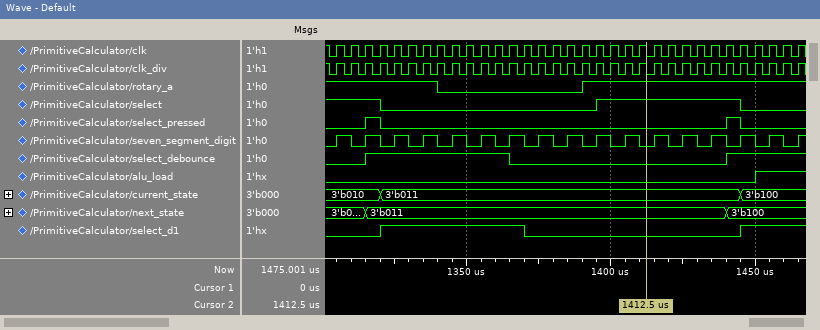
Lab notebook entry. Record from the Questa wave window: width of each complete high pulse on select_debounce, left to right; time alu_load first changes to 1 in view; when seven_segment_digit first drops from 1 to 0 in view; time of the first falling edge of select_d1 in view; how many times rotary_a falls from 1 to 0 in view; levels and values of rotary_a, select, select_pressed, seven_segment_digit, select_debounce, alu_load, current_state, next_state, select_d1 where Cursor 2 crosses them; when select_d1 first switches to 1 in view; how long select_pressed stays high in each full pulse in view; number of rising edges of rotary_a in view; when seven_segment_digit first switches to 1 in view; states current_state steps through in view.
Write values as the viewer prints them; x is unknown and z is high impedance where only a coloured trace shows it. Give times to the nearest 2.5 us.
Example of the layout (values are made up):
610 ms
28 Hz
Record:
50 us
1450 us
1310 us
1370 us
1
rotary_a=1, select=1, select_pressed=0, seven_segment_digit=0, select_debounce=0, alu_load=0, current_state=3'b011, next_state=3'b011, select_d1=0
1320 us
5 us, 5 us
1
1305 us
3'b010, 3'b011, 3'b100
